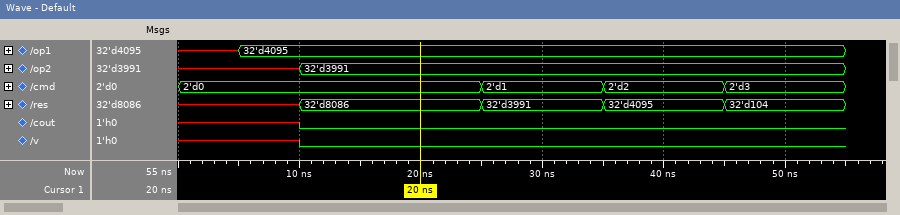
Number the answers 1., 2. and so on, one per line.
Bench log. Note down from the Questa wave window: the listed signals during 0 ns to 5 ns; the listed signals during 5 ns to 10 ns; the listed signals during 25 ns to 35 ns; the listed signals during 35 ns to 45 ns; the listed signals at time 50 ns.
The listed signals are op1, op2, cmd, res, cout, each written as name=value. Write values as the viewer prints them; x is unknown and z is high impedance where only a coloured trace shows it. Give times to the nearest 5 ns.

1. op1=x, op2=x, cmd=2'd0, res=x, cout=x
2. op1=32'd4095, op2=x, cmd=2'd0, res=x, cout=x
3. op1=32'd4095, op2=32'd3991, cmd=2'd1, res=32'd3991, cout=0
4. op1=32'd4095, op2=32'd3991, cmd=2'd2, res=32'd4095, cout=0
5. op1=32'd4095, op2=32'd3991, cmd=2'd3, res=32'd104, cout=0
